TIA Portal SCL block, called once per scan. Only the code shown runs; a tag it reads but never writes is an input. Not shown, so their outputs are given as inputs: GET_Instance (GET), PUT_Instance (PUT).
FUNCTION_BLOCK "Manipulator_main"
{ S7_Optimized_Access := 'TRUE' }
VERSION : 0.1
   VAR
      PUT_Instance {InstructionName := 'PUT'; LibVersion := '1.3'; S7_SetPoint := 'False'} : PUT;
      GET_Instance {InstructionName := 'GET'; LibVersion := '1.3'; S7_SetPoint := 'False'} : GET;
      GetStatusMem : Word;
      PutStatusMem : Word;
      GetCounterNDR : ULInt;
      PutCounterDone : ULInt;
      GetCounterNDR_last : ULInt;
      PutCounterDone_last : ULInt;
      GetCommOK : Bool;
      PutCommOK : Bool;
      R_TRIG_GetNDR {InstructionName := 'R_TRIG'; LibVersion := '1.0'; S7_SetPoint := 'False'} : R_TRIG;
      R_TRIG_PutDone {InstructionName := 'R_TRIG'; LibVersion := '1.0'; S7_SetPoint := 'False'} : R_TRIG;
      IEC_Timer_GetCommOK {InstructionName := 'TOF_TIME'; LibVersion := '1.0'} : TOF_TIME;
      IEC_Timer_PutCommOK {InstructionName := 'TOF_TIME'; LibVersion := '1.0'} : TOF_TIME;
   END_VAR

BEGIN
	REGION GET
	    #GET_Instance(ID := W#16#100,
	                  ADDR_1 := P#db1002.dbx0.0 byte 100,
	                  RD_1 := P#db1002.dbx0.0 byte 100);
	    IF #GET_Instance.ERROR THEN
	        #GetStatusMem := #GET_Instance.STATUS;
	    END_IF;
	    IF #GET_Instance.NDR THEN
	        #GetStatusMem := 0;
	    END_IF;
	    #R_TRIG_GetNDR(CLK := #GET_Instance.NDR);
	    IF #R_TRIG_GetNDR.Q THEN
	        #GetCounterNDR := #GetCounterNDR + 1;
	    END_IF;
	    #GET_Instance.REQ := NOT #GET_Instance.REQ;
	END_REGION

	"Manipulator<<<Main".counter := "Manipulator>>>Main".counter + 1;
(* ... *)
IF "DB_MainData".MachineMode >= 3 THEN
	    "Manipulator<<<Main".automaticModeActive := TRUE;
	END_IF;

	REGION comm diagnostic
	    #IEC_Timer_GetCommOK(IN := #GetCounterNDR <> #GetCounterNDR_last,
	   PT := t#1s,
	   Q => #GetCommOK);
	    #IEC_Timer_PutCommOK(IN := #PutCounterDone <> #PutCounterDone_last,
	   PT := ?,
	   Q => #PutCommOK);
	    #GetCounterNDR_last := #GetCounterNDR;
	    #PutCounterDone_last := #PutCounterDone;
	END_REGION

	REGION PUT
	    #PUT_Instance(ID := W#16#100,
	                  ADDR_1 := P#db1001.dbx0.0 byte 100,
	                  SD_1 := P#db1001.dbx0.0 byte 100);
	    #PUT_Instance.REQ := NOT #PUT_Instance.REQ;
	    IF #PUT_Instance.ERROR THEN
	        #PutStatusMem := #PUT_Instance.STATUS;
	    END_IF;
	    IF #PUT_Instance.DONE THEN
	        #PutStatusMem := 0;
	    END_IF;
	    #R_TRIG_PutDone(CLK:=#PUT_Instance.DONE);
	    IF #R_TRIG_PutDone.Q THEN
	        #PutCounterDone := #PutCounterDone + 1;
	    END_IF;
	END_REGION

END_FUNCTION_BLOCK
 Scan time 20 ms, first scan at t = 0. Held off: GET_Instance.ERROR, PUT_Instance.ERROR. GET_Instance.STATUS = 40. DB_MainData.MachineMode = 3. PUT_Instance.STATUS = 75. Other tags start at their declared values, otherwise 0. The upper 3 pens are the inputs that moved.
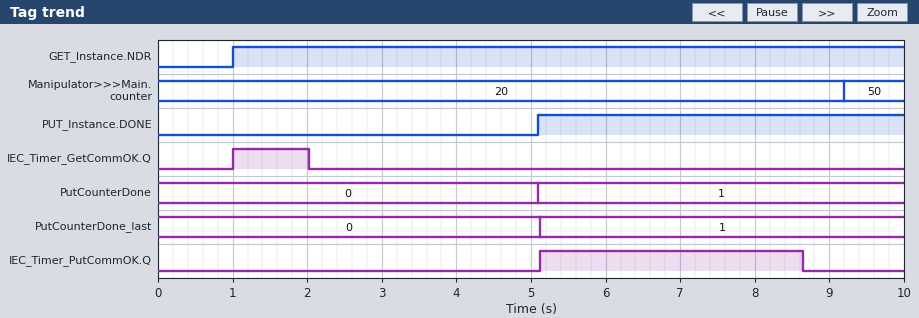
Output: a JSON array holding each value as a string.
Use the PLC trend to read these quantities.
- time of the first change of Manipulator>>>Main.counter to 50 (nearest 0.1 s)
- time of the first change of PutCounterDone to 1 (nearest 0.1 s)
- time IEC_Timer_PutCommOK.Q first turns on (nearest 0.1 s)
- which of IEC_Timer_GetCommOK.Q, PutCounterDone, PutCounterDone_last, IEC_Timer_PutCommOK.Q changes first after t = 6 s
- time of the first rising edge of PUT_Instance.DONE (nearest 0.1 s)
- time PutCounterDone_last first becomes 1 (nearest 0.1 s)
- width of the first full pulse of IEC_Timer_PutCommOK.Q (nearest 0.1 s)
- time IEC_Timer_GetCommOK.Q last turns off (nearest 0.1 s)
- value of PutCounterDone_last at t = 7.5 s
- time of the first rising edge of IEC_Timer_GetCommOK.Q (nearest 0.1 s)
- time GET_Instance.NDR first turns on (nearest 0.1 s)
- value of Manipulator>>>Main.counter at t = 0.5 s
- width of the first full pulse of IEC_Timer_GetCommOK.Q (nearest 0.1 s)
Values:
["9.2 s", "5.1 s", "5.1 s", "IEC_Timer_PutCommOK.Q", "5.1 s", "5.1 s", "3.5 s", "2.0 s", "1", "1.0 s", "1.0 s", "20", "1.0 s"]
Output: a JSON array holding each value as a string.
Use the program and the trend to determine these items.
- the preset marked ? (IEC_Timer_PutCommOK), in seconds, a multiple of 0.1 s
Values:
["3.5 s"]
